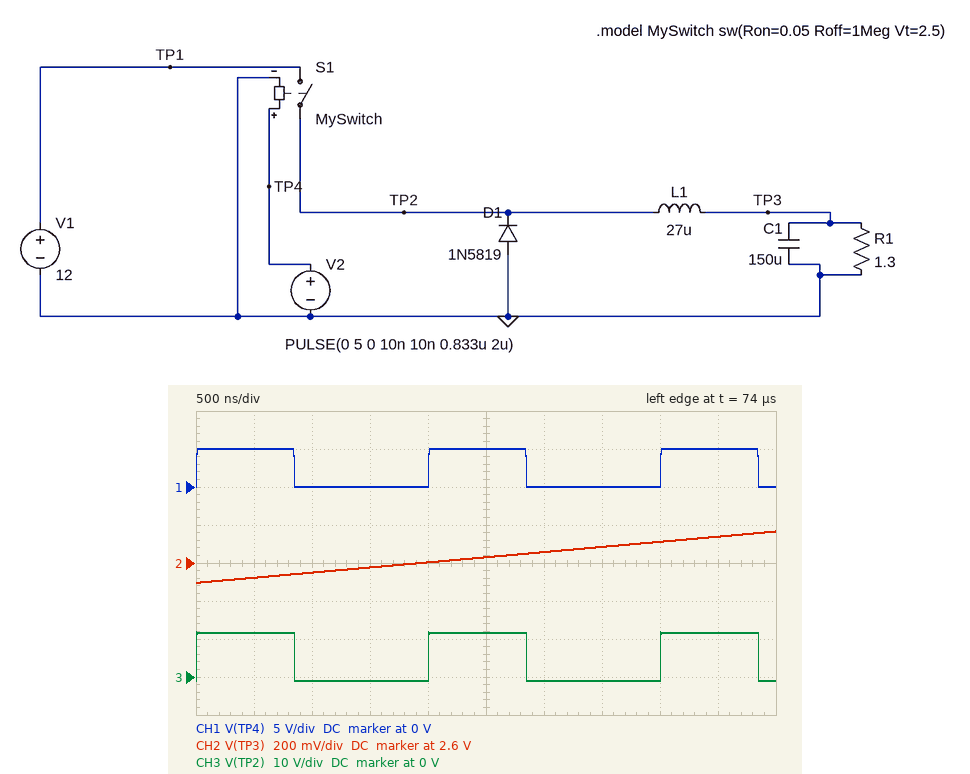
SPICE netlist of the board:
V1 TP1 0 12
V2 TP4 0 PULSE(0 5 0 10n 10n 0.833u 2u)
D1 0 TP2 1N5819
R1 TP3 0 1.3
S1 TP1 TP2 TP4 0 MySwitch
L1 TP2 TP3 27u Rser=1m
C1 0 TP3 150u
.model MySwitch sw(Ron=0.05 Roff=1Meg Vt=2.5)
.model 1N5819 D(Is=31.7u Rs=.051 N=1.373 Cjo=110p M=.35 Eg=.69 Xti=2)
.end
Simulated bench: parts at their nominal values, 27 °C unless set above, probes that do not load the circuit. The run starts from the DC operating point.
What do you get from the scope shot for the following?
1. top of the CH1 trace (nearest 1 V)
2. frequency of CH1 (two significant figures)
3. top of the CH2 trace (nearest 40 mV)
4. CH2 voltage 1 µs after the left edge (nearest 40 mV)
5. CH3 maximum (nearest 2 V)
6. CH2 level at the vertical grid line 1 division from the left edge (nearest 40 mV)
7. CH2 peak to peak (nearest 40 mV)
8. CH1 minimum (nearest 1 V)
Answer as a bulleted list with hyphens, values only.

- 5 V
- 500 kHz
- 2.76 V
- 2.56 V
- 12 V
- 2.52 V
- 280 mV
- 0 V
